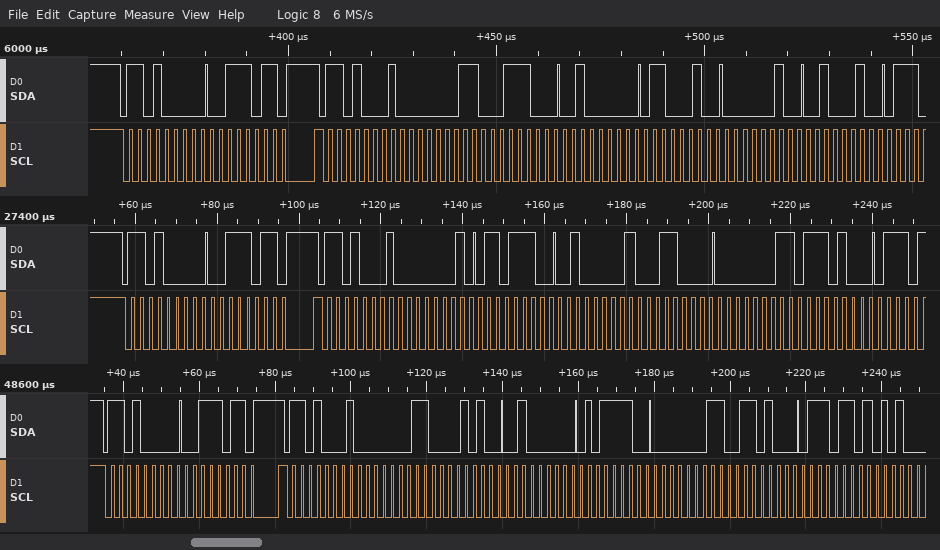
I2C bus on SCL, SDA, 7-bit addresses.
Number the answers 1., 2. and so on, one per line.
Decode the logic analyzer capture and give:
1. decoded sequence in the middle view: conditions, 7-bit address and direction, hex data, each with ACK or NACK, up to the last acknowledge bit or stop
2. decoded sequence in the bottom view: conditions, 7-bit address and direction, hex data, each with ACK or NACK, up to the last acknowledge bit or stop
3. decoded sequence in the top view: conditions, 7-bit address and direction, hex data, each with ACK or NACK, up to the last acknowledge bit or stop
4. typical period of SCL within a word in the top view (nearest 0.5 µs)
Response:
1. start, address 68 write ACK, 3B ACK, repeated start, address 68 read ACK, 02 ACK, DC ACK, 41 ACK, 30 ACK, 03 ACK, E8 ACK
2. start, address 68 write ACK, 3B ACK, repeated start, address 68 read ACK, 03 ACK, 14 ACK, 40 ACK, BC ACK, 03 ACK, 68 ACK, ED ACK
3. start, address 68 write ACK, 3B ACK, repeated start, address 68 read ACK, 03 ACK, 38 ACK, 40 ACK, C4 ACK, 04 ACK, 44 ACK
4. 2 µs
